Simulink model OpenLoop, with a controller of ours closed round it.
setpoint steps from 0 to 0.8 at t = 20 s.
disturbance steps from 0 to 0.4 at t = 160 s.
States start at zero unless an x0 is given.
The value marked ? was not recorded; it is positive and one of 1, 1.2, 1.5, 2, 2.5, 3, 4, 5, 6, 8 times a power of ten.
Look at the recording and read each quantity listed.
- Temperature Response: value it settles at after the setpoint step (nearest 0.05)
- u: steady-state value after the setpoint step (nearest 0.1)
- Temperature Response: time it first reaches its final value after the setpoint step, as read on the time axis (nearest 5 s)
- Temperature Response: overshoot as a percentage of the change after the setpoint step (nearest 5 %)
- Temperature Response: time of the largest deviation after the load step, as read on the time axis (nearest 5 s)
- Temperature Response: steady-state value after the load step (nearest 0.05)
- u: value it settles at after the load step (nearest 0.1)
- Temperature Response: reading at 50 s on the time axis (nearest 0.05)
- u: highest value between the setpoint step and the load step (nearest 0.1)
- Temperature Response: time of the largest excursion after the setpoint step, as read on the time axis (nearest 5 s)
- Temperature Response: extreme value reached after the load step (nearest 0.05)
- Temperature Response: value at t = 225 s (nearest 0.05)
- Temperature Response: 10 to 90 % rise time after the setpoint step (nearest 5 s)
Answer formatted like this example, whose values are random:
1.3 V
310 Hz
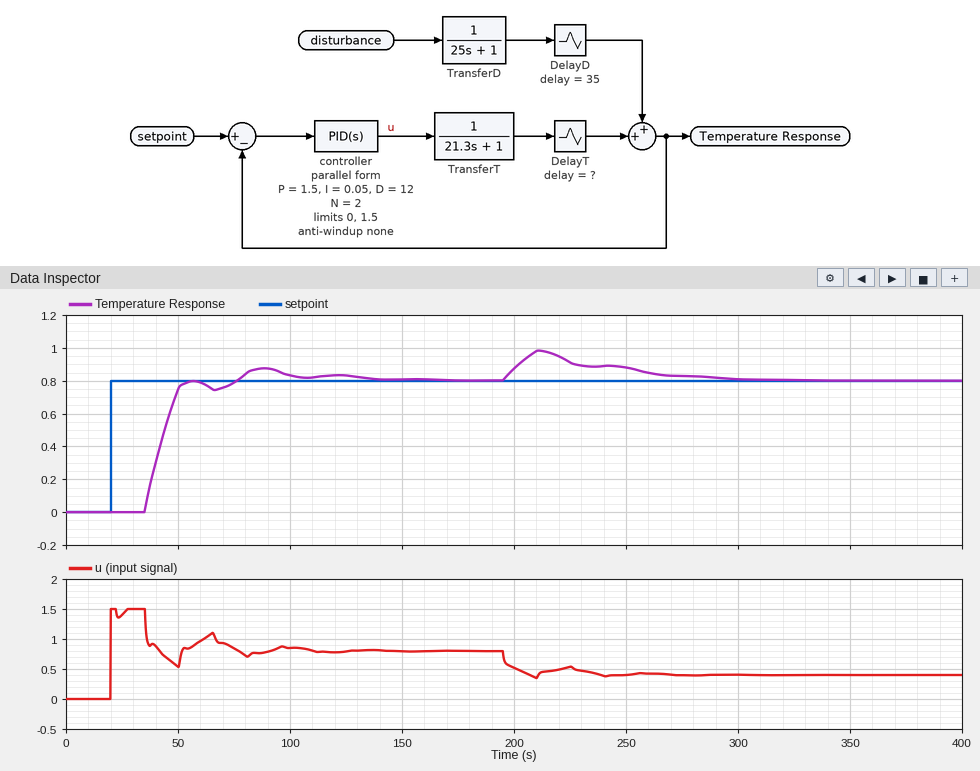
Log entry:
0.80
0.8
75 s
10 %
210 s
0.80
0.4
0.75
1.5
90 s
1.00
0.90
15 s
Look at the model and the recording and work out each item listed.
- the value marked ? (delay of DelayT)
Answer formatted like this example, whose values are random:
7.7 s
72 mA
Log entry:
15
